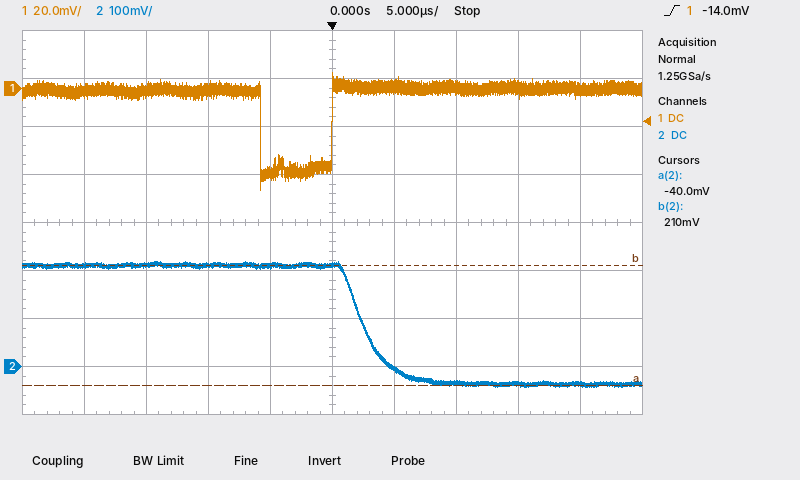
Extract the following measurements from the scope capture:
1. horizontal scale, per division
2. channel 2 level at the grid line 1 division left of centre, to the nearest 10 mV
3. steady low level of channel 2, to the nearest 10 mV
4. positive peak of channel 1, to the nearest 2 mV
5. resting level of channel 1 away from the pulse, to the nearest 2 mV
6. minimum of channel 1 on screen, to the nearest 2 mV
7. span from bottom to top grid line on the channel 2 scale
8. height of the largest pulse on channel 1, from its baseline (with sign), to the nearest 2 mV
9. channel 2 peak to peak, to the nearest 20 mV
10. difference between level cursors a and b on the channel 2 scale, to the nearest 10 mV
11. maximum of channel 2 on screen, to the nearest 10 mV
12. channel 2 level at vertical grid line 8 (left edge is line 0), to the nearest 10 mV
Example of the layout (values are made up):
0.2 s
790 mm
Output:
5 µs
210 mV
-40 mV
6 mV
0 mV
-42 mV
800 mV
-42 mV
260 mV
250 mV
220 mV
-40 mV
